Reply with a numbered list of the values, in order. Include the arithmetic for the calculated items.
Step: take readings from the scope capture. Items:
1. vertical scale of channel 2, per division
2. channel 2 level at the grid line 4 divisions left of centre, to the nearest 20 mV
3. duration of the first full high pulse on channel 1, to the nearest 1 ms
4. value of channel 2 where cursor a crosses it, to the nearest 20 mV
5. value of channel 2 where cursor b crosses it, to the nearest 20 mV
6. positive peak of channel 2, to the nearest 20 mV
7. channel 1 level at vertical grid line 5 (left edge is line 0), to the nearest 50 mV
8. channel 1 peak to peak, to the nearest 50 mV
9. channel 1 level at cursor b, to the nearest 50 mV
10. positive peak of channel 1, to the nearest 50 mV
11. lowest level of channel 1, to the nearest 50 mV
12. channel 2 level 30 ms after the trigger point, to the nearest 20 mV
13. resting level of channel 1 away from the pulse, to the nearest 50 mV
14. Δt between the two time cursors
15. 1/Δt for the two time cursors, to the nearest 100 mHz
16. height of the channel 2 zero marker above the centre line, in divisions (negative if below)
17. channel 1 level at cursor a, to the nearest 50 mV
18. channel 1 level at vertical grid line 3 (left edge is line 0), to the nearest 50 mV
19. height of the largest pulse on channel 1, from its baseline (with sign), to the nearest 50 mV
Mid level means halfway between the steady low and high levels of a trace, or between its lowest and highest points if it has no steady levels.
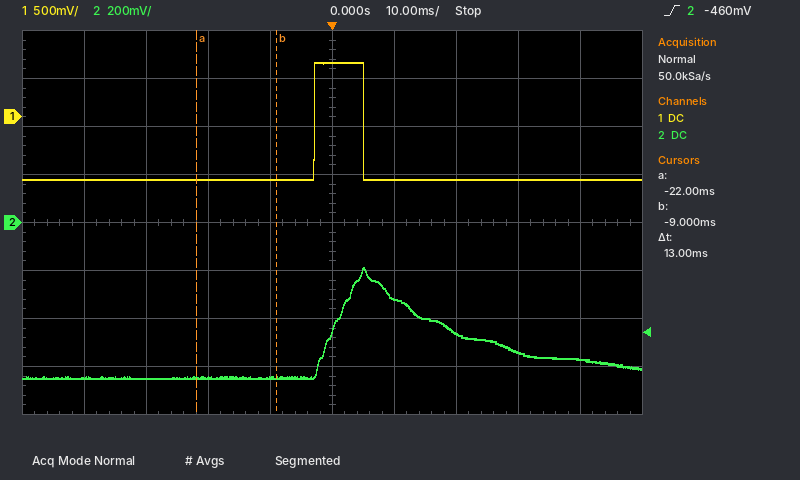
1. 200 mV
2. -640 mV
3. 8 ms
4. -640 mV
5. -640 mV
6. -180 mV
7. 550 mV
8. 550 mV − (-650 mV) = 1.20 V
9. -650 mV
10. 550 mV
11. -650 mV
12. -540 mV
13. -650 mV
14. 13 ms
15. 1 / 13 ms ≈ 76.9 Hz
16. 0.0 div
17. -650 mV
18. -650 mV
19. 550 mV − (-650 mV) = +1.20 V
